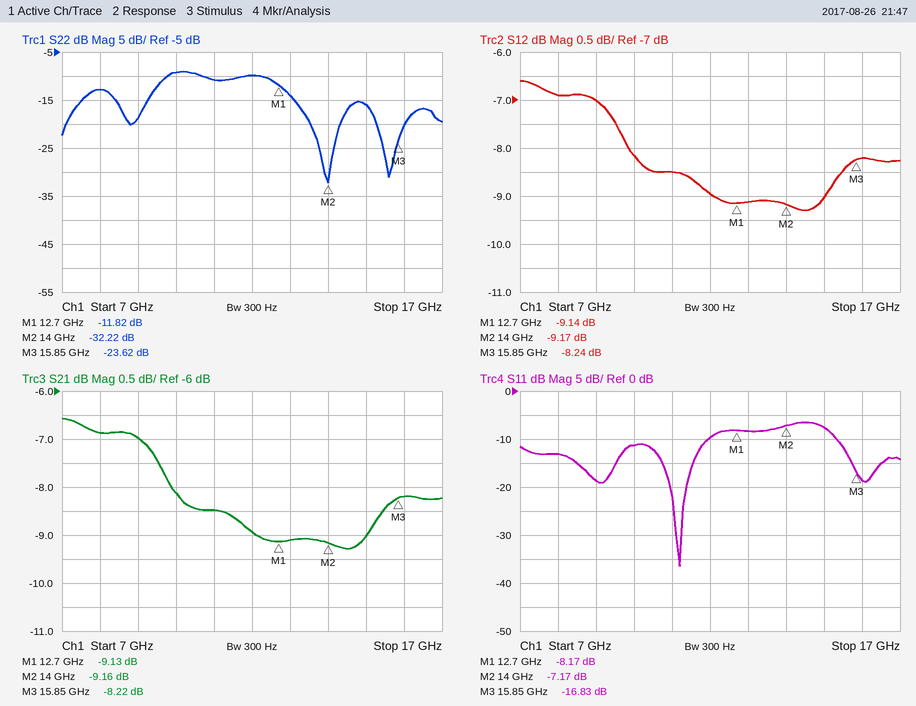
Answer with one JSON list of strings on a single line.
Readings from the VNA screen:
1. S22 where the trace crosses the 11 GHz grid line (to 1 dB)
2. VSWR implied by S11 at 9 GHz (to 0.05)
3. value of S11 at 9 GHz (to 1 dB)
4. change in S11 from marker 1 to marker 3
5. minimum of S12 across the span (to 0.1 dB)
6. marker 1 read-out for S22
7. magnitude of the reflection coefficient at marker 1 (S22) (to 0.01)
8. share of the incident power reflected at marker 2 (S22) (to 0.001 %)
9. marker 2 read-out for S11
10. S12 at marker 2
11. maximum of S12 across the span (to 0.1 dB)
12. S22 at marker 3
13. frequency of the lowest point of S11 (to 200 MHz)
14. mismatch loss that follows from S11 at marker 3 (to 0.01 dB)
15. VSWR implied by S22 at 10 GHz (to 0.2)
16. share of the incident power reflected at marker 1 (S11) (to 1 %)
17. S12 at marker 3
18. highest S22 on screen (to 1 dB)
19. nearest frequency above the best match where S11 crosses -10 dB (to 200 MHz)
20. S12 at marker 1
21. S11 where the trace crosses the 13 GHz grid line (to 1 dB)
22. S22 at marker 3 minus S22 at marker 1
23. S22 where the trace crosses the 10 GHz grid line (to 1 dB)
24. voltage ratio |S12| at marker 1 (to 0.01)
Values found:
["-11 dB", "1.25", "-19 dB", "-8.66 dB", "-9.3 dB", "-11.82 dB", "0.26", "0.060 %", "-7.17 dB", "-9.17 dB", "-6.6 dB", "-23.62 dB", "11.2 GHz", "0.09 dB", "2.0", "15 %", "-8.24 dB", "-9 dB", "12.0 GHz", "-9.14 dB", "-8 dB", "-11.80 dB", "-9 dB", "0.35"]
